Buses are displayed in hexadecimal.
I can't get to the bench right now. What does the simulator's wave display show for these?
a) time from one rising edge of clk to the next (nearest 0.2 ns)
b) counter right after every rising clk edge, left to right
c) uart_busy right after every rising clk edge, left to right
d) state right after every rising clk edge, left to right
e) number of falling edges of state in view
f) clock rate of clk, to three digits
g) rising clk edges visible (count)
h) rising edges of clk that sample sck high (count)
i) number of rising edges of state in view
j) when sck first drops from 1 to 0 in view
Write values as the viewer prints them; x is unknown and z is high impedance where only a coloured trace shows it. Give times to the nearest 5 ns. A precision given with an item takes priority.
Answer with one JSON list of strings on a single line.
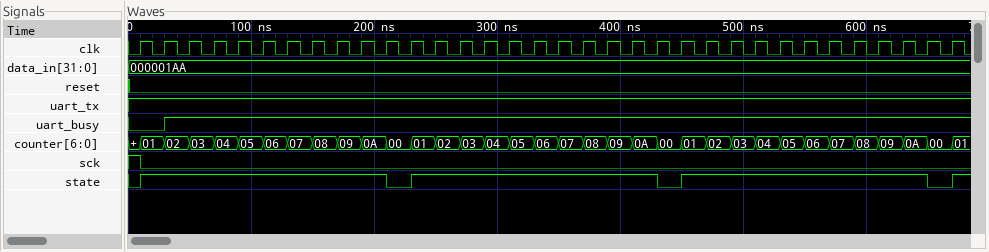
["20 ns", "01, 02, 03, 04, 05, 06, 07, 08, 09, 0A, 00, 01, 02, 03, 04, 05, 06, 07, 08, 09, 0A, 00, 01, 02, 03, 04, 05, 06, 07, 08, 09, 0A, 00, 01", "0 1 1 1 1 1 1 1 1 1 1 1 1 1 1 1 1 1 1 1 1 1 1 1 1 1 1 1 1 1 1 1 1 1", "1 1 1 1 1 1 1 1 1 1 0 1 1 1 1 1 1 1 1 1 1 0 1 1 1 1 1 1 1 1 1 1 0 1", "3", "50.0 MHz", "34", "1", "4", "10 ns"]
